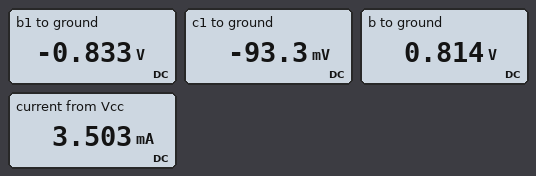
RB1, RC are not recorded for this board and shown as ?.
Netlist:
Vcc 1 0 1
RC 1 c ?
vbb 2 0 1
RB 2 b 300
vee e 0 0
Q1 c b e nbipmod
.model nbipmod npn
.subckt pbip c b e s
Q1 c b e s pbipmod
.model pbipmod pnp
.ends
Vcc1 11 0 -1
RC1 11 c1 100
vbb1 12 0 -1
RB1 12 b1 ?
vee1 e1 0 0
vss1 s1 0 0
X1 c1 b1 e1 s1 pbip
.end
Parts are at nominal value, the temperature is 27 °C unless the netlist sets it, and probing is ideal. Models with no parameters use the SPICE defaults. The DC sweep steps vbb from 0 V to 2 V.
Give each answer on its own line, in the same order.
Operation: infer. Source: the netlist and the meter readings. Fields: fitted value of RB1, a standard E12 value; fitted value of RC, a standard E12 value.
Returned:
470 Ω
270 Ω
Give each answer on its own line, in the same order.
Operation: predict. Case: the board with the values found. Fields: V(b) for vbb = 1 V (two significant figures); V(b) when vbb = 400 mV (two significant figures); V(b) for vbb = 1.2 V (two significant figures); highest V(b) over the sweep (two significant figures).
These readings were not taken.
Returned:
810 mV
400 mV
820 mV
840 mV
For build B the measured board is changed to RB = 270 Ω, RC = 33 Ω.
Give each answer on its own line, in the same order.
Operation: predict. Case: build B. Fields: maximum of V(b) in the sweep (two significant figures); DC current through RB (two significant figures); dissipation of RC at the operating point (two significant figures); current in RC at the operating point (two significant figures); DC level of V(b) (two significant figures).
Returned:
870 mV
520 µA
23 mW
27 mA
860 mV
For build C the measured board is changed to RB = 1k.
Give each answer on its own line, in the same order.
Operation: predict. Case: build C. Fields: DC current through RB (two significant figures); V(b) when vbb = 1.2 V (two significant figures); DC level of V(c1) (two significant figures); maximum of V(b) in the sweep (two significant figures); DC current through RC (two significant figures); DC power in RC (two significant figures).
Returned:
190 µA
810 mV
-93 mV
820 mV
3.4 mA
3.1 mW
